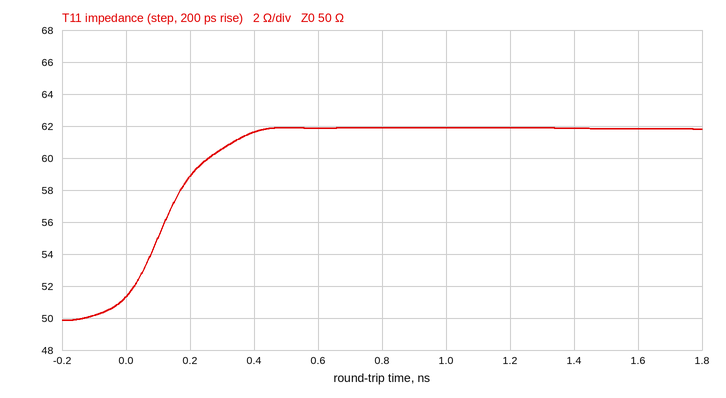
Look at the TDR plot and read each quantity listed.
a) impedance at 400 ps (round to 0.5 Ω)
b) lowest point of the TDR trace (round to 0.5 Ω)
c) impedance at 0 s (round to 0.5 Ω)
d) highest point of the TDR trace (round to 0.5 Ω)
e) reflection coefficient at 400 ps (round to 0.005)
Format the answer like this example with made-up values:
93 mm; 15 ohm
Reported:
61.5 Ω; 50.0 Ω; 51.5 Ω; 62.0 Ω; +0.105
